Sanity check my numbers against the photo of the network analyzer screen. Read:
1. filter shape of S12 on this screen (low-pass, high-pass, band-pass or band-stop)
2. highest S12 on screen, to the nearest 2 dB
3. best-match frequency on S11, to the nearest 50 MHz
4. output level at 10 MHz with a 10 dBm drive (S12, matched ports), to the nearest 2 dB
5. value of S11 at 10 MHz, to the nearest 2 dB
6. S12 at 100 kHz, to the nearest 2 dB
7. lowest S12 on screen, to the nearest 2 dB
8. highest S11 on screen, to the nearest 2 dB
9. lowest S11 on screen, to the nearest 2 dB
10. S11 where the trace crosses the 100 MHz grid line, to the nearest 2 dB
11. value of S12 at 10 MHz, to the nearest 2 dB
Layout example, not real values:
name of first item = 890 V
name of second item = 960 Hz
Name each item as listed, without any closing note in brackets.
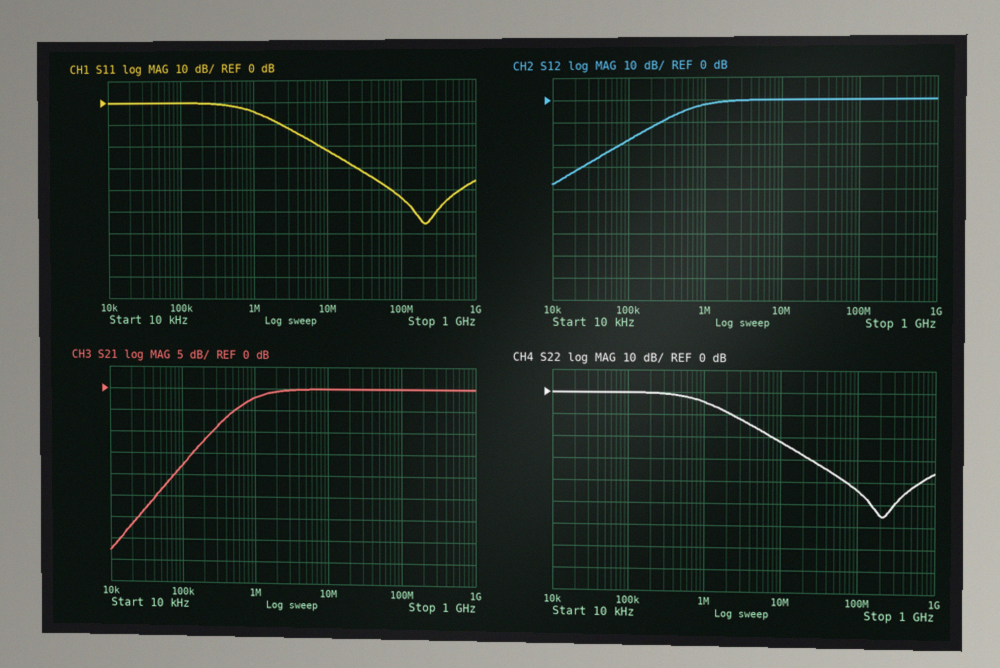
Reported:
filter shape of S12 on this screen = high-pass
highest S12 on screen, to the nearest 2 dB = 0 dB
best-match frequency on S11, to the nearest 50 MHz = 200 MHz
output level at 10 MHz with a 10 dBm drive (S12, matched ports), to the nearest 2 dB = 10 dBm
value of S11 at 10 MHz, to the nearest 2 dB = -22 dB
S12 at 100 kHz, to the nearest 2 dB = -18 dB
lowest S12 on screen, to the nearest 2 dB = -38 dB
highest S11 on screen, to the nearest 2 dB = 0 dB
lowest S11 on screen, to the nearest 2 dB = -56 dB
S11 where the trace crosses the 100 MHz grid line, to the nearest 2 dB = -44 dB
value of S12 at 10 MHz, to the nearest 2 dB = 0 dB
